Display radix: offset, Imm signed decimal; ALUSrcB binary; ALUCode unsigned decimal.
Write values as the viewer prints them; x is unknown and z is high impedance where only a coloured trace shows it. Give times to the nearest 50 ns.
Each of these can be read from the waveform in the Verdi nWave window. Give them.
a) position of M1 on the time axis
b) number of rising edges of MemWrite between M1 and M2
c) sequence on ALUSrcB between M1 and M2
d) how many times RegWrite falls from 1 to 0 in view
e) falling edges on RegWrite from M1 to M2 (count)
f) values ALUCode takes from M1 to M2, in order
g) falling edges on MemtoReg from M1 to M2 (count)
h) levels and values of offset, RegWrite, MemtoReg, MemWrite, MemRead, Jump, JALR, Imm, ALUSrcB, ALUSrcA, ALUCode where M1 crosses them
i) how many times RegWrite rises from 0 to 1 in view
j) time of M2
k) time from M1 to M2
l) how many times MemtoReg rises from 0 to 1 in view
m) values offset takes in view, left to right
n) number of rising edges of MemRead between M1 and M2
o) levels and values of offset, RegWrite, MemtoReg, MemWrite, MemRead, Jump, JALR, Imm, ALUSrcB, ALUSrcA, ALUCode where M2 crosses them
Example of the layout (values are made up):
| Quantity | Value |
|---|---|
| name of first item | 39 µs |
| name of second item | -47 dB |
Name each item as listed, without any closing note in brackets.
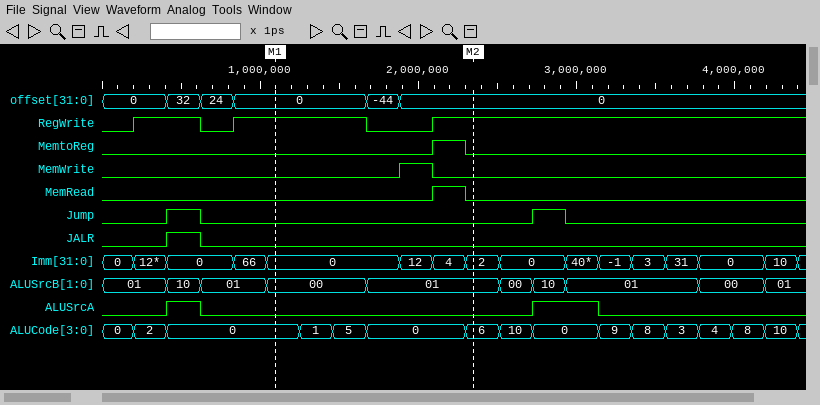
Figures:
| Quantity | Value |
|---|---|
| position of M1 on the time axis | 1100 ns |
| number of rising edges of MemWrite between M1 and M2 | 1 |
| sequence on ALUSrcB between M1 and M2 | 00, 01 |
| how many times RegWrite falls from 1 to 0 in view | 2 |
| falling edges on RegWrite from M1 to M2 | 1 |
| values ALUCode takes from M1 to M2, in order | 0, 1, 5, 0, 6 |
| falling edges on MemtoReg from M1 to M2 | 1 |
| levels and values of offset, RegWrite, MemtoReg, MemWrite, MemRead, Jump, JALR, Imm, ALUSrcB, ALUSrcA, ALUCode where M1 crosses them | offset=0, RegWrite=1, MemtoReg=0, MemWrite=0, MemRead=0, Jump=0, JALR=0, Imm=0, ALUSrcB=00, ALUSrcA=0, ALUCode=0 |
| how many times RegWrite rises from 0 to 1 in view | 3 |
| time of M2 | 2350 ns |
| time from M1 to M2 | 1250 ns |
| how many times MemtoReg rises from 0 to 1 in view | 1 |
| values offset takes in view, left to right | 0, 32, 24, 0, -44, 0 |
| number of rising edges of MemRead between M1 and M2 | 1 |
| levels and values of offset, RegWrite, MemtoReg, MemWrite, MemRead, Jump, JALR, Imm, ALUSrcB, ALUSrcA, ALUCode where M2 crosses them | offset=0, RegWrite=1, MemtoReg=0, MemWrite=0, MemRead=0, Jump=0, JALR=0, Imm=2, ALUSrcB=01, ALUSrcA=0, ALUCode=6 |
